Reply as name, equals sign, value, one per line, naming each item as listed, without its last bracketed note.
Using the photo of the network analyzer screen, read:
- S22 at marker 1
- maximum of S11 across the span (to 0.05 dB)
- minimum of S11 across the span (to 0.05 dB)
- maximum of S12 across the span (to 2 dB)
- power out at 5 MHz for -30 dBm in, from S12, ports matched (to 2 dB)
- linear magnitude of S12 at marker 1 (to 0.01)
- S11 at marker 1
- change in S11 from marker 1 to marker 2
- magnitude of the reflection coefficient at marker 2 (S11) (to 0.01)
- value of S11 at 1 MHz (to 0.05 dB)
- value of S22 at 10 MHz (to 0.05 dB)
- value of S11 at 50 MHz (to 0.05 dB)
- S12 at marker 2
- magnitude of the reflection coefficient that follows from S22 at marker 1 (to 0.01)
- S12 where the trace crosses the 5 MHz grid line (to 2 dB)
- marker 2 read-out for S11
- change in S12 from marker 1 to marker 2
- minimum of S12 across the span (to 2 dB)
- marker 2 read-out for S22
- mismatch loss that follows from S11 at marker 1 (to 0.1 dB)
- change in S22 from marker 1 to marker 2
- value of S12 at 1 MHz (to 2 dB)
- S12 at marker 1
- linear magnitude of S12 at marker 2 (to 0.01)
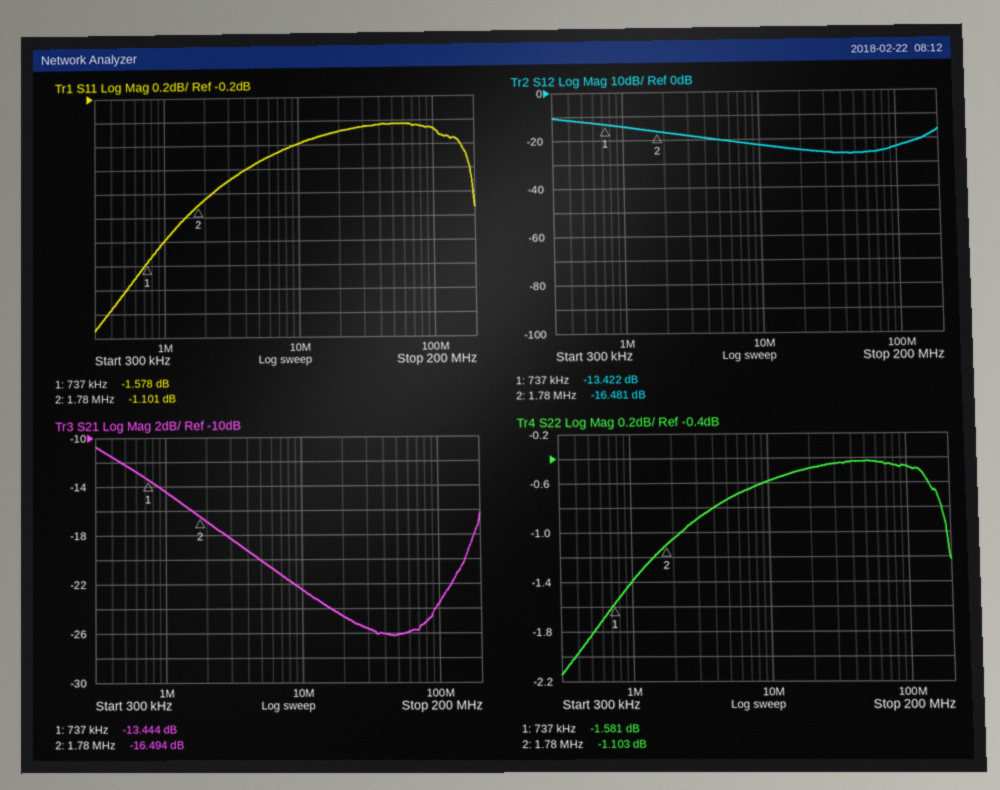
S22 at marker 1 = -1.581 dB
maximum of S11 across the span = -0.45 dB
minimum of S11 across the span = -2.15 dB
maximum of S12 across the span = -10 dB
power out at 5 MHz for -30 dBm in, from S12, ports matched = -50 dBm
linear magnitude of S12 at marker 1 = 0.21
S11 at marker 1 = -1.578 dB
change in S11 from marker 1 to marker 2 = 0.477 dB
magnitude of the reflection coefficient at marker 2 (S11) = 0.88
value of S11 at 1 MHz = -1.40 dB
value of S22 at 10 MHz = -0.60 dB
value of S11 at 50 MHz = -0.45 dB
S12 at marker 2 = -16.481 dB
magnitude of the reflection coefficient that follows from S22 at marker 1 = 0.83
S12 where the trace crosses the 5 MHz grid line = -20 dB
marker 2 read-out for S11 = -1.101 dB
change in S12 from marker 1 to marker 2 = -3.059 dB
minimum of S12 across the span = -26 dB
marker 2 read-out for S22 = -1.103 dB
mismatch loss that follows from S11 at marker 1 = 5.2 dB
change in S22 from marker 1 to marker 2 = 0.478 dB
value of S12 at 1 MHz = -14 dB
S12 at marker 1 = -13.422 dB
linear magnitude of S12 at marker 2 = 0.15
